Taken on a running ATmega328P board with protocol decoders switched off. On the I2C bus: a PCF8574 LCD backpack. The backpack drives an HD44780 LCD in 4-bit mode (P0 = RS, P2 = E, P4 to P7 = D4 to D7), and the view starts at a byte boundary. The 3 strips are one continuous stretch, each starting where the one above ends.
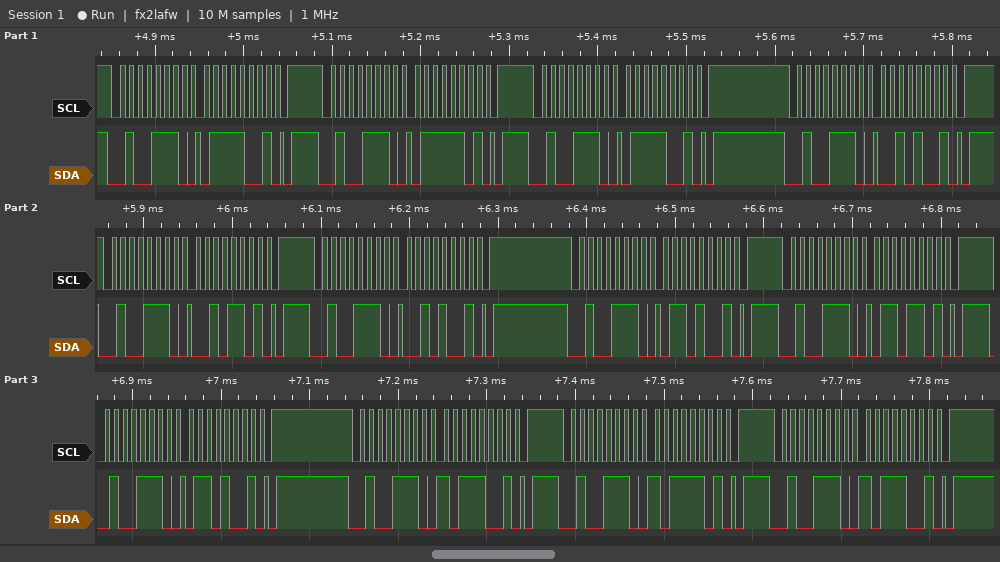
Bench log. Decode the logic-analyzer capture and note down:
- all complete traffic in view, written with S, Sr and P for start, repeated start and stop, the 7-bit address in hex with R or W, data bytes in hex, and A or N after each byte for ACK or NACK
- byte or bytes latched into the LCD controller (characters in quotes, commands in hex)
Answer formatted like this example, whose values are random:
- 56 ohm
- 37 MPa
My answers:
- S 27W A 79 A P S 27W A 7D A P S 27W A 79 A P S 27W A 29 A P S 27W A 2D A P S 27W A 29 A P S 27W A 69 A P S 27W A 6D A P S 27W A 69 A P S 27W A B9 A P S 27W A BD A P S 27W A B9 A P
- 'r' 'k'
